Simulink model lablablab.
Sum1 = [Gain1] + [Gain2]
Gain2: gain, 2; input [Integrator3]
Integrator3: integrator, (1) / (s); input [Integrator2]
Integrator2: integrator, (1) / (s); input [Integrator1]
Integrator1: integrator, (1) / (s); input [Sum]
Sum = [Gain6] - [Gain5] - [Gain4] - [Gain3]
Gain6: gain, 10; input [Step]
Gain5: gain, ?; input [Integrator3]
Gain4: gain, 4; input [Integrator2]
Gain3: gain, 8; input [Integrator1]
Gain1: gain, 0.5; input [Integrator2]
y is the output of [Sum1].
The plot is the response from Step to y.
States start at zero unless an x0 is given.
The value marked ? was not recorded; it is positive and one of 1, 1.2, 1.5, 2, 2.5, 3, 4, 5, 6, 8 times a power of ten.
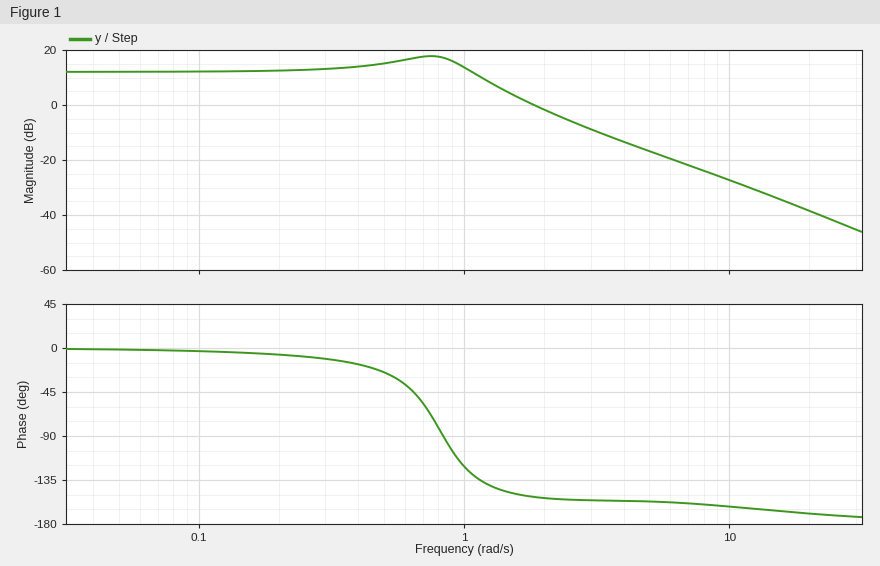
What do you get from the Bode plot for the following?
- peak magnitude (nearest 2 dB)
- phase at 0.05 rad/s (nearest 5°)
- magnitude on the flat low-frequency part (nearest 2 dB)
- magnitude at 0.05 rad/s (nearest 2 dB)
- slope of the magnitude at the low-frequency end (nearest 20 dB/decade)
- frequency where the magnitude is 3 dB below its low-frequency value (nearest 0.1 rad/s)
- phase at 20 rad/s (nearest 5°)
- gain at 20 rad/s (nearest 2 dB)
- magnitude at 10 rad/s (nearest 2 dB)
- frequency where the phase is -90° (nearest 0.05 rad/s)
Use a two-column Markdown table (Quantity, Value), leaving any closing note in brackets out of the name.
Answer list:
| Quantity | Value |
|---|---|
| peak magnitude | 18 dB |
| phase at 0.05 rad/s | 0° |
| magnitude on the flat low-frequency part | 12 dB |
| magnitude at 0.05 rad/s | 12 dB |
| slope of the magnitude at the low-frequency end | 0 dB/decade |
| frequency where the magnitude is 3 dB below its low-frequency value | 1.2 rad/s |
| phase at 20 rad/s | -170° |
| gain at 20 rad/s | -38 dB |
| magnitude at 10 rad/s | -28 dB |
| frequency where the phase is -90° | 0.85 rad/s |
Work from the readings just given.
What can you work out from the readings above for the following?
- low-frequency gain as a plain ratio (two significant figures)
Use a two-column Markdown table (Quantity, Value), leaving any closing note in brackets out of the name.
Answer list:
| Quantity | Value |
|---|---|
| low-frequency gain as a plain ratio | 4.0 |
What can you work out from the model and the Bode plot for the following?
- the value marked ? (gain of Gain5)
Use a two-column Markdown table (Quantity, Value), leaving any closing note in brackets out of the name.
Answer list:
| Quantity | Value |
|---|---|
| the value marked ? | 5 |
